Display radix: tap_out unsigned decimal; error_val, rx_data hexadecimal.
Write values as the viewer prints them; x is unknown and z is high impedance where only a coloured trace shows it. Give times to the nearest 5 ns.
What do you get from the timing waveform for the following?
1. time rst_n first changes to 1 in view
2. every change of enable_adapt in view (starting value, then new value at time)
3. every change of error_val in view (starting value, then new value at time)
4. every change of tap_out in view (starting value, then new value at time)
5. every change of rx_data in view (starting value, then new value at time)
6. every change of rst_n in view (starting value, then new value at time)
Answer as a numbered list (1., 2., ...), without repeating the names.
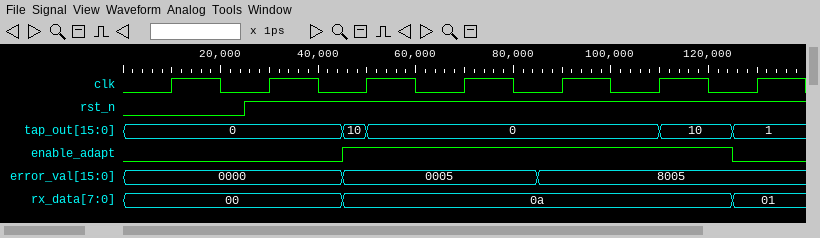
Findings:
1. 25 ns
2. 0, 1 at 45 ns, 0 at 125 ns
3. 0000, 0005 at 45 ns, 8005 at 85 ns
4. 0, 10 at 45 ns, 0 at 50 ns, 10 at 110 ns, 1 at 125 ns
5. 00, 0a at 45 ns, 01 at 125 ns
6. 0, 1 at 25 ns
